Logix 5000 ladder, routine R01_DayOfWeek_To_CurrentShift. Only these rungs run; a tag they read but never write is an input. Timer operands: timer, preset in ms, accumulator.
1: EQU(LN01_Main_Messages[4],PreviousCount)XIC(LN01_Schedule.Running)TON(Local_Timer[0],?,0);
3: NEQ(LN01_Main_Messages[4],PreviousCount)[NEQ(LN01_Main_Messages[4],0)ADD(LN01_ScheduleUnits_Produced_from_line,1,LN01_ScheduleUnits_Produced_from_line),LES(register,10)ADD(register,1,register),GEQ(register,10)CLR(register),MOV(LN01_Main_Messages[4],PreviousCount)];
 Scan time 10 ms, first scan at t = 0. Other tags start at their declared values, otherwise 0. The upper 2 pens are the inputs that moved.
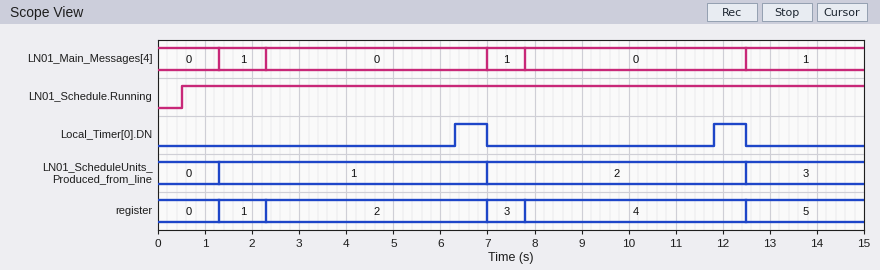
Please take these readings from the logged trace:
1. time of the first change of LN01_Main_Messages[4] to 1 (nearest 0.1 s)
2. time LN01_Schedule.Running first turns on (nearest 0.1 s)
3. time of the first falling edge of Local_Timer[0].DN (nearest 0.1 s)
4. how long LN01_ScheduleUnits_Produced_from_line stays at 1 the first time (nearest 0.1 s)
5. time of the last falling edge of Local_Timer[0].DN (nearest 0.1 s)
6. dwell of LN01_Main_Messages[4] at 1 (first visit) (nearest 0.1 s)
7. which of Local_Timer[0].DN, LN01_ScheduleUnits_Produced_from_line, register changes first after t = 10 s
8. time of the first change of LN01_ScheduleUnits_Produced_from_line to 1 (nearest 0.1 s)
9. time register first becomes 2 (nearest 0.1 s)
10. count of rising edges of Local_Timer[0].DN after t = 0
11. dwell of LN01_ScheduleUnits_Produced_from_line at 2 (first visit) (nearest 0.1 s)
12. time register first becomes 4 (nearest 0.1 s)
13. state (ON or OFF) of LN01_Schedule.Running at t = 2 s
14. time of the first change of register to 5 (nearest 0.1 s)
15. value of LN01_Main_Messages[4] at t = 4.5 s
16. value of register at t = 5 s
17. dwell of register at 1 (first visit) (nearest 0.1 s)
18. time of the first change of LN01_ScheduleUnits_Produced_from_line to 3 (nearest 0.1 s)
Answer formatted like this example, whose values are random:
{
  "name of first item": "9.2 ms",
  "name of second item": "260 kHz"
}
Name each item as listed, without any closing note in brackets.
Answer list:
{
  "time of the first change of LN01_Main_Messages[4] to 1": "1.3 s",
  "time LN01_Schedule.Running first turns on": "0.5 s",
  "time of the first falling edge of Local_Timer[0].DN": "7.0 s",
  "how long LN01_ScheduleUnits_Produced_from_line stays at 1 the first time": "5.7 s",
  "time of the last falling edge of Local_Timer[0].DN": "12.5 s",
  "dwell of LN01_Main_Messages[4] at 1 (first visit)": "1.0 s",
  "which of Local_Timer[0].DN, LN01_ScheduleUnits_Produced_from_line, register changes first after t = 10 s": "Local_Timer[0].DN",
  "time of the first change of LN01_ScheduleUnits_Produced_from_line to 1": "1.3 s",
  "time register first becomes 2": "2.3 s",
  "count of rising edges of Local_Timer[0].DN after t = 0": "2",
  "dwell of LN01_ScheduleUnits_Produced_from_line at 2 (first visit)": "5.5 s",
  "time register first becomes 4": "7.8 s",
  "state (ON or OFF) of LN01_Schedule.Running at t = 2 s": "ON",
  "time of the first change of register to 5": "12.5 s",
  "value of LN01_Main_Messages[4] at t = 4.5 s": "0",
  "value of register at t = 5 s": "2",
  "dwell of register at 1 (first visit)": "1.0 s",
  "time of the first change of LN01_ScheduleUnits_Produced_from_line to 3": "12.5 s"
}
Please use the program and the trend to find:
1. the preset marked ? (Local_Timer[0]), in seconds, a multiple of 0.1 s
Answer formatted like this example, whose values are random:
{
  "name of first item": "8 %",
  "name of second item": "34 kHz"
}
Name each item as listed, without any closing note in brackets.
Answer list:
{
  "the preset marked ? (Local_Timer[0]), in seconds, a multiple of 0.1 s": "4.0 s"
}
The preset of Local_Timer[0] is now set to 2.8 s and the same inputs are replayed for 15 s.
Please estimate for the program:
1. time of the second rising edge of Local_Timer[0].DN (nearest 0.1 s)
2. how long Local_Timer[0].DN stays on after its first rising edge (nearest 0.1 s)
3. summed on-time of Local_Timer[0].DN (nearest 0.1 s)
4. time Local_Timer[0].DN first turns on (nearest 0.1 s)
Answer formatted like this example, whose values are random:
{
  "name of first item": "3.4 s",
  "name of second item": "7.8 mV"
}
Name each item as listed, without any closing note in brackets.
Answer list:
{
  "time of the second rising edge of Local_Timer[0].DN": "10.6 s",
  "how long Local_Timer[0].DN stays on after its first rising edge": "1.9 s",
  "summed on-time of Local_Timer[0].DN": "3.8 s",
  "time Local_Timer[0].DN first turns on": "5.1 s"
}
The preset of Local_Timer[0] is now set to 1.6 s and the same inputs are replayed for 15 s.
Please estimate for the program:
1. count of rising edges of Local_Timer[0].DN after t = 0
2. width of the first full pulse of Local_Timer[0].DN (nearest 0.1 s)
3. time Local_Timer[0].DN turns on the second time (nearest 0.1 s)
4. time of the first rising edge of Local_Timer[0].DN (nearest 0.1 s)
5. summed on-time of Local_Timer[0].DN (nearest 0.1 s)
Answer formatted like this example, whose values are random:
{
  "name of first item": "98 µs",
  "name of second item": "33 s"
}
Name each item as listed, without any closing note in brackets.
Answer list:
{
  "count of rising edges of Local_Timer[0].DN after t = 0": "3",
  "width of the first full pulse of Local_Timer[0].DN": "3.1 s",
  "time Local_Timer[0].DN turns on the second time": "9.4 s",
  "time of the first rising edge of Local_Timer[0].DN": "3.9 s",
  "summed on-time of Local_Timer[0].DN": "7.1 s"
}
